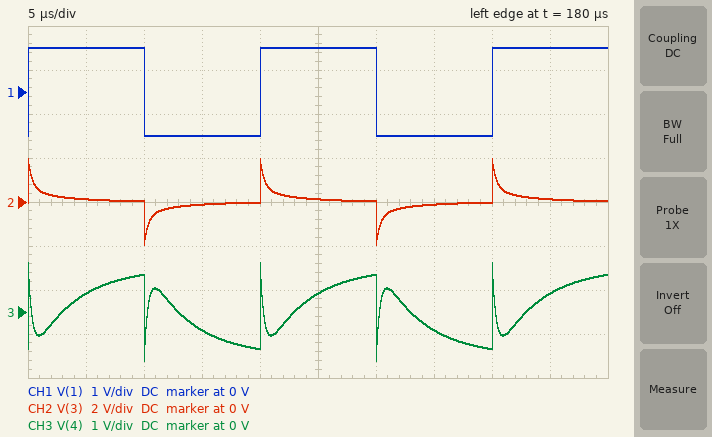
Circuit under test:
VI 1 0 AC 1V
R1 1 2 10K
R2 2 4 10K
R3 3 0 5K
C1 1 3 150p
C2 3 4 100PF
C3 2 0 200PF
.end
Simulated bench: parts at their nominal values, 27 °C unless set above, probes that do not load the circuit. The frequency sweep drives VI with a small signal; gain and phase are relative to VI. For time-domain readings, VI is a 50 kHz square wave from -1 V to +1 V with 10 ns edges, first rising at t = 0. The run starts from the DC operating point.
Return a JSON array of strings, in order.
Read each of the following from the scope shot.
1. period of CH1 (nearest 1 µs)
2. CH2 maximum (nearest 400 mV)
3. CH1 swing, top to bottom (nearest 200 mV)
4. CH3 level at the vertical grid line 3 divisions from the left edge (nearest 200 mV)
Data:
["20 µs", "2.0 V", "2.0 V", "-400 mV"]
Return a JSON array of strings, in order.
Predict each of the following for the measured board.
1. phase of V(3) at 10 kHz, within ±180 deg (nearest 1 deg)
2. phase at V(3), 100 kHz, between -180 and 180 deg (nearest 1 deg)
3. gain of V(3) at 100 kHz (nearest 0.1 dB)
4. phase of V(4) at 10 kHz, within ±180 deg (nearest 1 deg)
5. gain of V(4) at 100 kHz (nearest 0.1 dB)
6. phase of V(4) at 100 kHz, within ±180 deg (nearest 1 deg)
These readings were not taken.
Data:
["80 deg", "46 deg", "-8.2 dB", "-14 deg", "-14.9 dB", "-70 deg"]
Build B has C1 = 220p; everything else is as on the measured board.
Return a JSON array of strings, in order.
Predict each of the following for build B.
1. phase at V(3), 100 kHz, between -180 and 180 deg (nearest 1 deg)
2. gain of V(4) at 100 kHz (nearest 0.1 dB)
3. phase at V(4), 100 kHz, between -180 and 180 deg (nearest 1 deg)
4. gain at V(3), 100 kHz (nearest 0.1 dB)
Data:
["42 deg", "-17.4 dB", "-49 deg", "-5.9 dB"]
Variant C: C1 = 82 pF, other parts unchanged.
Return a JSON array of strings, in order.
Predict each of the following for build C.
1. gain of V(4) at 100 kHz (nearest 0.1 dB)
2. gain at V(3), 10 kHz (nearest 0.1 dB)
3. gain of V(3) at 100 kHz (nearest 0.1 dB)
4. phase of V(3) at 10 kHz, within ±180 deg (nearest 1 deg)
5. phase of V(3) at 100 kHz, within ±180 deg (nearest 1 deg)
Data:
["-11.8 dB", "-25.1 dB", "-12.1 dB", "79 deg", "44 deg"]
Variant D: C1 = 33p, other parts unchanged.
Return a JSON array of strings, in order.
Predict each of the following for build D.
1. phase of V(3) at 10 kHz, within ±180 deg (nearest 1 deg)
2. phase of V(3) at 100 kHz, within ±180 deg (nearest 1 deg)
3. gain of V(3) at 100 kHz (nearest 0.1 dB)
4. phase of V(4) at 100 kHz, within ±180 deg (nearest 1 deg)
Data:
["77 deg", "29 deg", "-16.6 dB", "-78 deg"]
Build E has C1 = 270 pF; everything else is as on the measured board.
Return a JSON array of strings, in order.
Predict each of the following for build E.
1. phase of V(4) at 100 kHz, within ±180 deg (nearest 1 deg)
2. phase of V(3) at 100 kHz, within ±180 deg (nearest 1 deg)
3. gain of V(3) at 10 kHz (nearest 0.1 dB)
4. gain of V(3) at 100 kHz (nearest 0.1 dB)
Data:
["-30 deg", "39 deg", "-18.9 dB", "-4.8 dB"]
